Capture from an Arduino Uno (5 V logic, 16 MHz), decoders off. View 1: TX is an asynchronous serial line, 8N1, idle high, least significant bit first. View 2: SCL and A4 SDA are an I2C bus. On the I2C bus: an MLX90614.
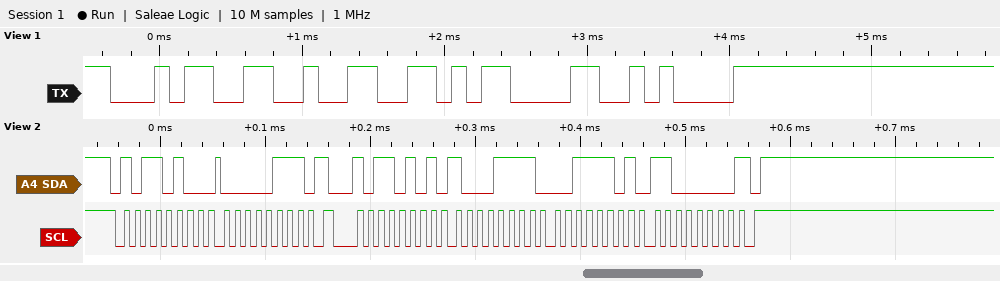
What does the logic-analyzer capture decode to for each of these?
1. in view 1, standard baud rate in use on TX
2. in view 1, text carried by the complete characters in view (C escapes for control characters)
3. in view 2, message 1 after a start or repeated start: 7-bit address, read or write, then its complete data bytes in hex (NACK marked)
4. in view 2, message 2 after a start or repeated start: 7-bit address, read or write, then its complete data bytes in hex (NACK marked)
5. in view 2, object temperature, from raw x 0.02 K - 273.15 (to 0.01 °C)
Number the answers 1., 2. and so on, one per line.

1. 9600 baud
2. "42\r\n"
3. 0x5A write: 07
4. 0x5A read: 8F 3D C0 NACK
5. 42.03 °C
